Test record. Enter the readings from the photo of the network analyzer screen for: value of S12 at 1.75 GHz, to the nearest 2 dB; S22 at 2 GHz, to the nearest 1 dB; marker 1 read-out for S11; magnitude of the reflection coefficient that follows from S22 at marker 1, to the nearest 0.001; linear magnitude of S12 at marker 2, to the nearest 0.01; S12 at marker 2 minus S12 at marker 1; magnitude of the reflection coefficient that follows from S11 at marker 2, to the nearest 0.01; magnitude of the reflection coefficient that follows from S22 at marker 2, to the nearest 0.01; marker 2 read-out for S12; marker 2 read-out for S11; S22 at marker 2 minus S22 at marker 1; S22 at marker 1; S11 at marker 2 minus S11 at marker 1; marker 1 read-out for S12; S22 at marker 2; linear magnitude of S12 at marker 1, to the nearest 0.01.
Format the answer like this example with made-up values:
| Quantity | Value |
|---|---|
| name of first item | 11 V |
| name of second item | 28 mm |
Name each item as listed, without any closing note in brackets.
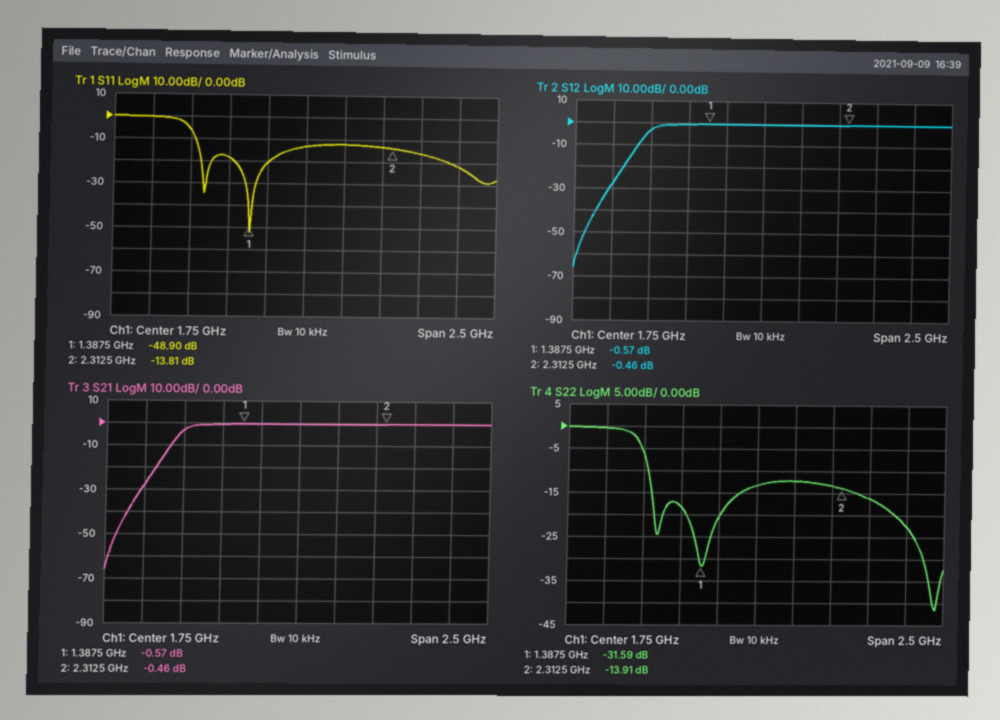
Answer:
| Quantity | Value |
|---|---|
| value of S12 at 1.75 GHz, to the nearest 2 dB | 0 dB |
| S22 at 2 GHz, to the nearest 1 dB | -12 dB |
| marker 1 read-out for S11 | -48.90 dB |
| magnitude of the reflection coefficient that follows from S22 at marker 1, to the nearest 0.001 | 0.026 |
| linear magnitude of S12 at marker 2, to the nearest 0.01 | 0.95 |
| S12 at marker 2 minus S12 at marker 1 | 0.11 dB |
| magnitude of the reflection coefficient that follows from S11 at marker 2, to the nearest 0.01 | 0.20 |
| magnitude of the reflection coefficient that follows from S22 at marker 2, to the nearest 0.01 | 0.20 |
| marker 2 read-out for S12 | -0.46 dB |
| marker 2 read-out for S11 | -13.81 dB |
| S22 at marker 2 minus S22 at marker 1 | 17.68 dB |
| S22 at marker 1 | -31.59 dB |
| S11 at marker 2 minus S11 at marker 1 | 35.09 dB |
| marker 1 read-out for S12 | -0.57 dB |
| S22 at marker 2 | -13.91 dB |
| linear magnitude of S12 at marker 1, to the nearest 0.01 | 0.94 |
